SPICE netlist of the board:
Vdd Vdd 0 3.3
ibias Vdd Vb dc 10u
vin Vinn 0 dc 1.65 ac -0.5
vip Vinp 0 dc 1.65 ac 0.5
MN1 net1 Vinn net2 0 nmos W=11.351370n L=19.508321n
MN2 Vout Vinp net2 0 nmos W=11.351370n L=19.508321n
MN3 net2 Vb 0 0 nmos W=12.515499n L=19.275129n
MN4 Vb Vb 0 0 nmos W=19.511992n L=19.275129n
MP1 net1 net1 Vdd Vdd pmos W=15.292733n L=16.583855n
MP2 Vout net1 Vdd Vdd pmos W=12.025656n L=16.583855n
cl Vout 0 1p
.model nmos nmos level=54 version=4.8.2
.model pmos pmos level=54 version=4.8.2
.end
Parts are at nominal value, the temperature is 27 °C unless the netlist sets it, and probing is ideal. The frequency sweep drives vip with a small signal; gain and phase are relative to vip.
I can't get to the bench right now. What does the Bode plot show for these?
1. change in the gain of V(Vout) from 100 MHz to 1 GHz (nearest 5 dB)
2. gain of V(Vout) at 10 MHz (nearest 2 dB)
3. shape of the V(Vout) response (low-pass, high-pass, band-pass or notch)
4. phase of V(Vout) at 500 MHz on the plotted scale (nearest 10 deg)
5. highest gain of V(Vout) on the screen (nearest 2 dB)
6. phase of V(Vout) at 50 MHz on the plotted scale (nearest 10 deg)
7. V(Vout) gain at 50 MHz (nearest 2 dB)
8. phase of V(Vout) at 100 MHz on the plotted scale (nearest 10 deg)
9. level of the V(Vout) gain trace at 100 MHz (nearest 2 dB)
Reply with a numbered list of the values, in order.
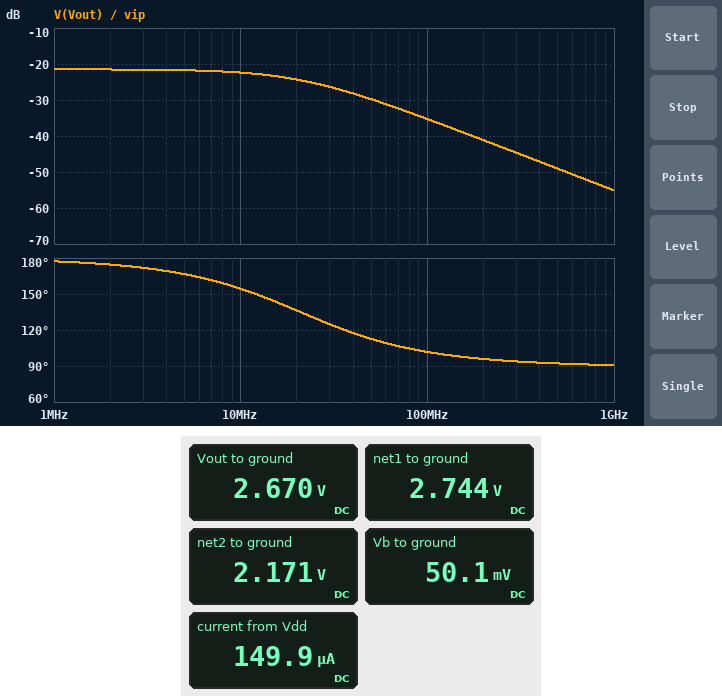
1. -20 dB
2. -22 dB
3. low-pass
4. 90 deg
5. -22 dB
6. 110 deg
7. -30 dB
8. 100 deg
9. -36 dB
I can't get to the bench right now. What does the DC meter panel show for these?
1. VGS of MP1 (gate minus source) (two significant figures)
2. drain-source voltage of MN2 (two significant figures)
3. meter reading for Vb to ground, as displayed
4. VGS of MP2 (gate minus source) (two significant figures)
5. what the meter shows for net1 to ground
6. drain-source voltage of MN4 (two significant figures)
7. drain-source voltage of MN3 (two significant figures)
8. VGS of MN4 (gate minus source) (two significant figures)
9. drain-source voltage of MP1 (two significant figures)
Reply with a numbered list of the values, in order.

1. -560 mV
2. 500 mV
3. 50.1 mV
4. -560 mV
5. 2.744 V
6. 50 mV
7. 2.2 V
8. 50 mV
9. -560 mV
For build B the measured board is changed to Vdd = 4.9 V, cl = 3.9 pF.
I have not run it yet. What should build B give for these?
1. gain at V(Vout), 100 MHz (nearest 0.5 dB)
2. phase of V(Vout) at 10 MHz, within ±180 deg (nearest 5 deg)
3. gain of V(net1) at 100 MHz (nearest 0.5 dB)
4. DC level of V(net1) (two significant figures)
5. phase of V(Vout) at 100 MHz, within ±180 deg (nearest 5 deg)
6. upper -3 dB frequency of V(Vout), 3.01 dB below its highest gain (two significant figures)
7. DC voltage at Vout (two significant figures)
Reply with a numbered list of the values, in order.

1. -45.0 dB
2. 115 deg
3. -27.0 dB
4. 3.9 V
5. 95 deg
6. 5.1 MHz
7. 3.8 V
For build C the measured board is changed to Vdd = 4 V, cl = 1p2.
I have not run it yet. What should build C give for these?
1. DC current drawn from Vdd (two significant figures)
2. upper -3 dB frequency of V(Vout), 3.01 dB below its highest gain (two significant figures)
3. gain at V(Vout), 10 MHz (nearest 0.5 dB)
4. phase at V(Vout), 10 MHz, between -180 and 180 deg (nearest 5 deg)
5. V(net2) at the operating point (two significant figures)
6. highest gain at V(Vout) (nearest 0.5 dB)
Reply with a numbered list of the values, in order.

1. 190 µA
2. 17 MHz
3. -21.0 dB
4. 150 deg
5. 2.3 V
6. -20.0 dB
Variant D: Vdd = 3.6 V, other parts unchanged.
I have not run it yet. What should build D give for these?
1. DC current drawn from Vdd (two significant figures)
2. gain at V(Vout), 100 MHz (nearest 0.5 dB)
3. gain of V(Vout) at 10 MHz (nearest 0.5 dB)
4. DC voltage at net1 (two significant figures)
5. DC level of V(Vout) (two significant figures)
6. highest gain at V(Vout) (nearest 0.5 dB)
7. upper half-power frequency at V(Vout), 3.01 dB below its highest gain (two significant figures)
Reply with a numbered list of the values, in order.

1. 170 µA
2. -34.5 dB
3. -21.5 dB
4. 3.0 V
5. 2.9 V
6. -20.5 dB
7. 20 MHz
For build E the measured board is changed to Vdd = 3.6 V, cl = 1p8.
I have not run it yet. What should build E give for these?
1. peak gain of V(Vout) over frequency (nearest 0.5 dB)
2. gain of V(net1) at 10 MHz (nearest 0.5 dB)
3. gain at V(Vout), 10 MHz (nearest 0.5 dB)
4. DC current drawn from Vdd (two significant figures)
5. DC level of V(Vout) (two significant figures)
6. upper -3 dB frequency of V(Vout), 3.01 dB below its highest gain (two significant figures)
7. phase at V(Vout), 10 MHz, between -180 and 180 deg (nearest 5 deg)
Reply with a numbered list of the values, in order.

1. -20.5 dB
2. -27.0 dB
3. -23.0 dB
4. 170 µA
5. 2.9 V
6. 11 MHz
7. 140 deg
